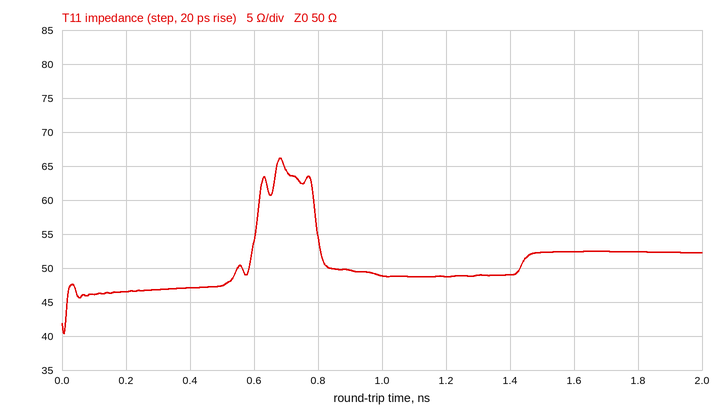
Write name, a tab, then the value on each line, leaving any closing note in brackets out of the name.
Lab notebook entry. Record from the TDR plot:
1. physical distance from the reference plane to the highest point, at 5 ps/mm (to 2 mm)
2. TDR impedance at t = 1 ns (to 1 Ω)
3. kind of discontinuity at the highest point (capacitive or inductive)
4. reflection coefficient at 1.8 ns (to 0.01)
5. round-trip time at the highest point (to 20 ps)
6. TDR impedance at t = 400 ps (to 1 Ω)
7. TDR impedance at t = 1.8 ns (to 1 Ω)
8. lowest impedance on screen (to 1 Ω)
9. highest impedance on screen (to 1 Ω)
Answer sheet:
physical distance from the reference plane to the highest point, at 5 ps/mm	68 mm
TDR impedance at t = 1 ns	49 Ω
kind of discontinuity at the highest point	inductive
reflection coefficient at 1.8 ns	+0.02
round-trip time at the highest point	680 ps
TDR impedance at t = 400 ps	47 Ω
TDR impedance at t = 1.8 ns	52 Ω
lowest impedance on screen	40 Ω
highest impedance on screen	66 Ω
